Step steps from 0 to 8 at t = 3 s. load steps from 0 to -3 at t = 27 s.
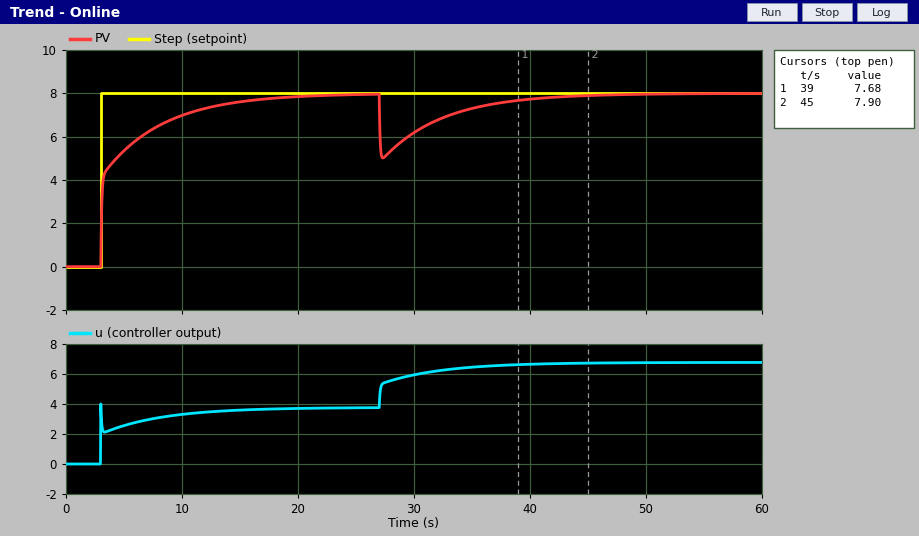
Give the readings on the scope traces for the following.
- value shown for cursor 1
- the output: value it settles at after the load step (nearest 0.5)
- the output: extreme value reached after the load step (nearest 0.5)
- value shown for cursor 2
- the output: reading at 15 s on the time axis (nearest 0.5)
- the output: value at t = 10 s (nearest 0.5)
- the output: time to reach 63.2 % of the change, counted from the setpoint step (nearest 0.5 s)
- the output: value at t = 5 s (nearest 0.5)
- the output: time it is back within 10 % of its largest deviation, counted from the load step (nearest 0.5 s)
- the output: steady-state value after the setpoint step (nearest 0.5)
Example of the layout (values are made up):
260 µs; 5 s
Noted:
7.68; 8.0; 5.0; 7.90; 7.5; 7.0; 1.5 s; 5.5; 12.5 s; 8.0
